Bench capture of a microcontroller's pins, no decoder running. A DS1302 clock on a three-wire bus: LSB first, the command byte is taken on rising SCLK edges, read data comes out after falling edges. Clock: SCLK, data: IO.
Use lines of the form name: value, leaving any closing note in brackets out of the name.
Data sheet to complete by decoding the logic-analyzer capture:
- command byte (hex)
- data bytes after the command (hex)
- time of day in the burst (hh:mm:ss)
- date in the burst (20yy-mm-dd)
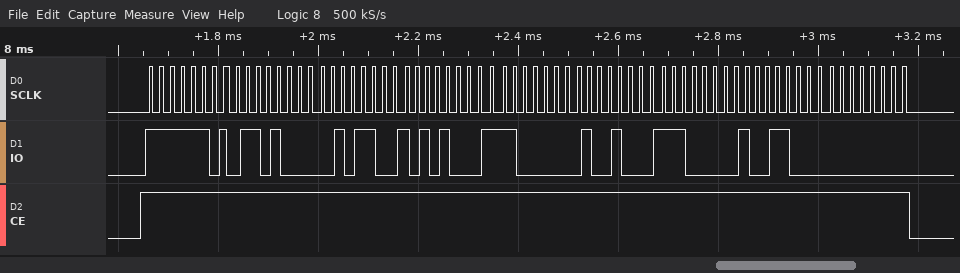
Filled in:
command byte: 0xBF
data bytes after the command: 16 34 15 07 12 07 19 00
time of day in the burst: 15:34:16
date in the burst: 2019-12-07
